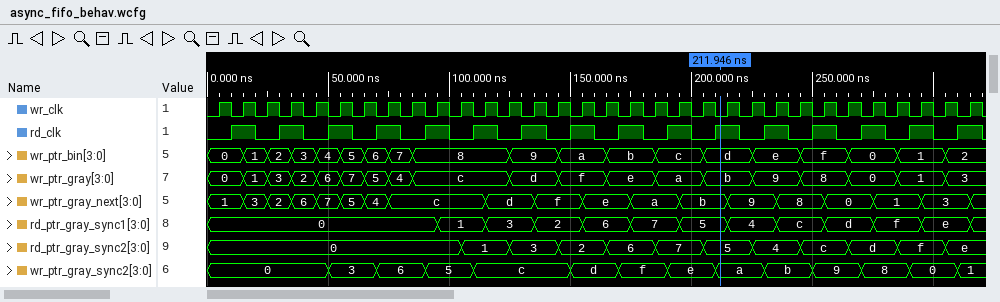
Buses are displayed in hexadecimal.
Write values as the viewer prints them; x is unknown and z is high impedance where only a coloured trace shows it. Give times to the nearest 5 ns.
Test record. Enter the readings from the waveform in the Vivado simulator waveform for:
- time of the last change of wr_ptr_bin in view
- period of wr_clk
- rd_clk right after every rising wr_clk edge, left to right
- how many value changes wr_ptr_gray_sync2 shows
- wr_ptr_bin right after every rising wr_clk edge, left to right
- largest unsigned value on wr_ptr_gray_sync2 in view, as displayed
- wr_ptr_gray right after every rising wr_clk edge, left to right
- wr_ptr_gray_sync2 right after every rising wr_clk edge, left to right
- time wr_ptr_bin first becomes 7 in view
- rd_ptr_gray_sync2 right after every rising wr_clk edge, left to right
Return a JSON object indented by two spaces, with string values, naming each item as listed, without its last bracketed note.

{
  "time of the last change of wr_ptr_bin in view": "305 ns",
  "period of wr_clk": "10 ns",
  "rd_clk right after every rising wr_clk edge, left to right": "0 1 0 1 0 1 0 1 0 1 0 1 0 1 0 1 0 1 0 1 0 1 0 1 0 1 0 1 0 1 0 1",
  "how many value changes wr_ptr_gray_sync2 shows": "13",
  "wr_ptr_bin right after every rising wr_clk edge, left to right": "0, 1, 2, 3, 4, 5, 6, 7, 8, 8, 8, 8, 9, 9, a, a, b, b, c, c, d, d, e, e, f, f, 0, 0, 1, 1, 2, 2",
  "largest unsigned value on wr_ptr_gray_sync2 in view, as displayed": "f",
  "wr_ptr_gray right after every rising wr_clk edge, left to right": "0, 1, 3, 2, 6, 7, 5, 4, c, c, c, c, d, d, f, f, e, e, a, a, b, b, 9, 9, 8, 8, 0, 0, 1, 1, 3, 3",
  "wr_ptr_gray_sync2 right after every rising wr_clk edge, left to right": "0, 0, 0, 0, 0, 3, 3, 6, 6, 5, 5, c, c, c, c, d, d, f, f, e, e, a, a, b, b, 9, 9, 8, 8, 0, 0, 1",
  "time wr_ptr_bin first becomes 7 in view": "75 ns",
  "rd_ptr_gray_sync2 right after every rising wr_clk edge, left to right": "0, 0, 0, 0, 0, 0, 0, 0, 0, 0, 1, 1, 3, 3, 2, 2, 6, 6, 7, 7, 5, 5, 4, 4, c, c, d, d, f, f, e, e"
}
